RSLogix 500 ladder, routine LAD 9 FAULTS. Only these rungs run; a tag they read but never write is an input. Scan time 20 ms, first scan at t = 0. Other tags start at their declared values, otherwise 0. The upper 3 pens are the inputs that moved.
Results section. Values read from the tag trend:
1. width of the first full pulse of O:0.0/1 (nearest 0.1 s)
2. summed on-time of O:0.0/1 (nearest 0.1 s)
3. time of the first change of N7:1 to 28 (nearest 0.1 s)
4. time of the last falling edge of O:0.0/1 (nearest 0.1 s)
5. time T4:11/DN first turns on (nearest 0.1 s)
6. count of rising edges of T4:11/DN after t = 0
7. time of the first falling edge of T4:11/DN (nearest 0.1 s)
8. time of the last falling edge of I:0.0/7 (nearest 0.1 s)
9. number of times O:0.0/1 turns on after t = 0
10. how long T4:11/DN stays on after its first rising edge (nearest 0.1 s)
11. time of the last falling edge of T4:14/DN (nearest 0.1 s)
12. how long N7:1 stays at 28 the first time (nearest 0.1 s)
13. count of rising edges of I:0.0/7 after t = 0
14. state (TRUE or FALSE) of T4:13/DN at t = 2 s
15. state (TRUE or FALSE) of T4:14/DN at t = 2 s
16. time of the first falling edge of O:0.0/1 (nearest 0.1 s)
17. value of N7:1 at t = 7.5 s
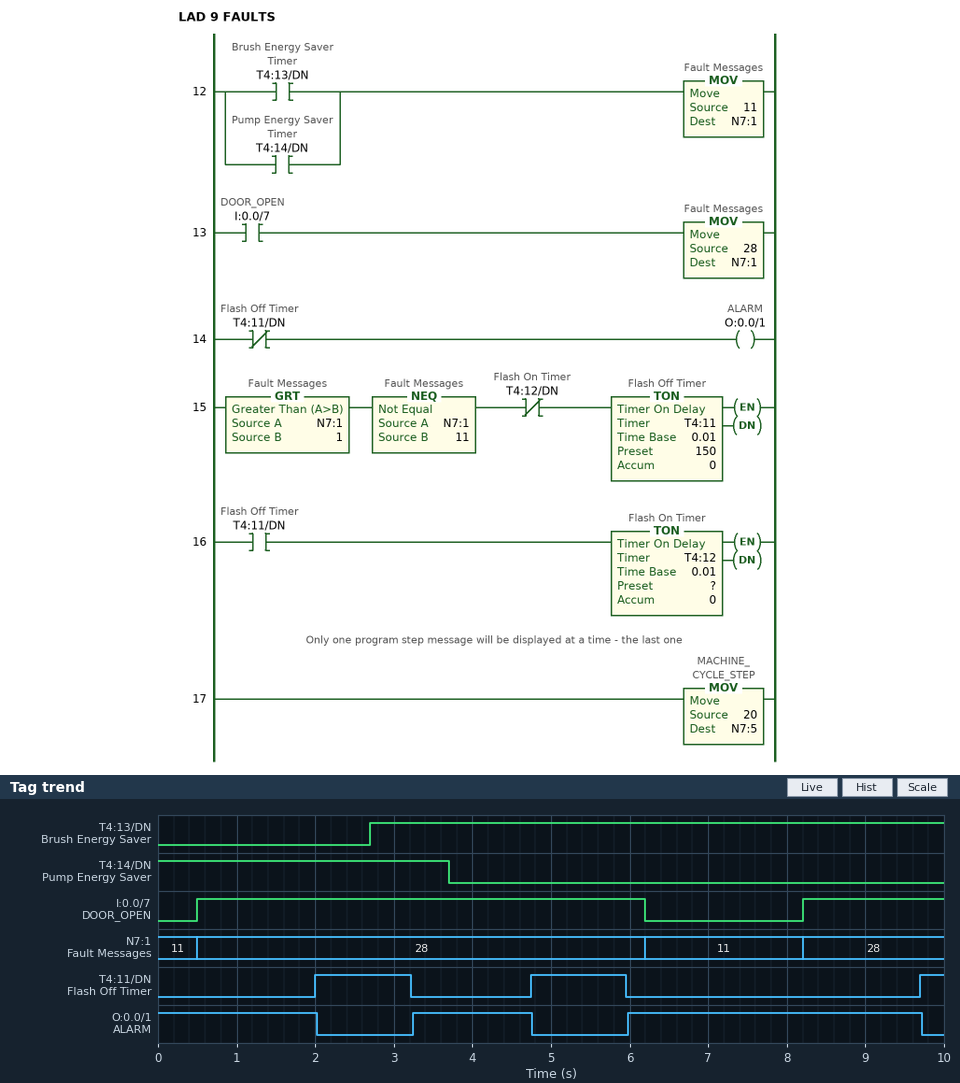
1.5 s
7.3 s
0.5 s
9.7 s
2.0 s
3
3.2 s
6.2 s
2
1.2 s
3.7 s
5.7 s
2
FALSE
TRUE
2.0 s
11
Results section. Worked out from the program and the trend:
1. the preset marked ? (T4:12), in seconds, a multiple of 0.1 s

1.2 s
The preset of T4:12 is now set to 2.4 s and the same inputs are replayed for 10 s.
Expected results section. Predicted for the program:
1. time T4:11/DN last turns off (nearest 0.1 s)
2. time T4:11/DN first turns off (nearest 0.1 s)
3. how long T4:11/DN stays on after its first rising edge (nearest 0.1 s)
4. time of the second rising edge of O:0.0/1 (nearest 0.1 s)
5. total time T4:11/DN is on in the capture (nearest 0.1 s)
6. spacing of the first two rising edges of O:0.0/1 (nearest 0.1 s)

6.2 s
4.4 s
2.4 s
6.2 s
3.0 s
1.8 s
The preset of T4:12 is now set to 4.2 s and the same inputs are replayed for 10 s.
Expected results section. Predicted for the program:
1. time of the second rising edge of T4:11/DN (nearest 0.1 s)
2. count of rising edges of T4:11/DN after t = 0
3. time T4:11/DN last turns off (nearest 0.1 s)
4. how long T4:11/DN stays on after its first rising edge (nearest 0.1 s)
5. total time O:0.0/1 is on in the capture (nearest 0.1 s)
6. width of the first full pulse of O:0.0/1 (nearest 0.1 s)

9.7 s
2
6.2 s
4.2 s
5.5 s
3.5 s
